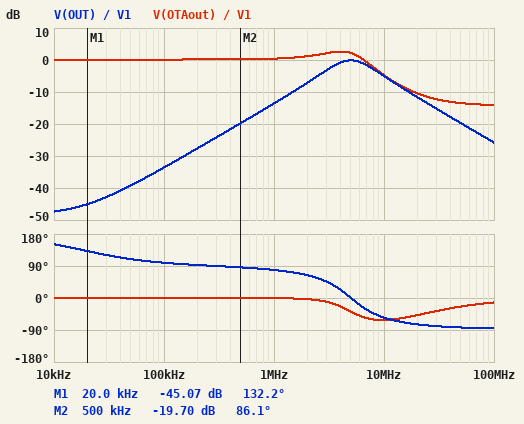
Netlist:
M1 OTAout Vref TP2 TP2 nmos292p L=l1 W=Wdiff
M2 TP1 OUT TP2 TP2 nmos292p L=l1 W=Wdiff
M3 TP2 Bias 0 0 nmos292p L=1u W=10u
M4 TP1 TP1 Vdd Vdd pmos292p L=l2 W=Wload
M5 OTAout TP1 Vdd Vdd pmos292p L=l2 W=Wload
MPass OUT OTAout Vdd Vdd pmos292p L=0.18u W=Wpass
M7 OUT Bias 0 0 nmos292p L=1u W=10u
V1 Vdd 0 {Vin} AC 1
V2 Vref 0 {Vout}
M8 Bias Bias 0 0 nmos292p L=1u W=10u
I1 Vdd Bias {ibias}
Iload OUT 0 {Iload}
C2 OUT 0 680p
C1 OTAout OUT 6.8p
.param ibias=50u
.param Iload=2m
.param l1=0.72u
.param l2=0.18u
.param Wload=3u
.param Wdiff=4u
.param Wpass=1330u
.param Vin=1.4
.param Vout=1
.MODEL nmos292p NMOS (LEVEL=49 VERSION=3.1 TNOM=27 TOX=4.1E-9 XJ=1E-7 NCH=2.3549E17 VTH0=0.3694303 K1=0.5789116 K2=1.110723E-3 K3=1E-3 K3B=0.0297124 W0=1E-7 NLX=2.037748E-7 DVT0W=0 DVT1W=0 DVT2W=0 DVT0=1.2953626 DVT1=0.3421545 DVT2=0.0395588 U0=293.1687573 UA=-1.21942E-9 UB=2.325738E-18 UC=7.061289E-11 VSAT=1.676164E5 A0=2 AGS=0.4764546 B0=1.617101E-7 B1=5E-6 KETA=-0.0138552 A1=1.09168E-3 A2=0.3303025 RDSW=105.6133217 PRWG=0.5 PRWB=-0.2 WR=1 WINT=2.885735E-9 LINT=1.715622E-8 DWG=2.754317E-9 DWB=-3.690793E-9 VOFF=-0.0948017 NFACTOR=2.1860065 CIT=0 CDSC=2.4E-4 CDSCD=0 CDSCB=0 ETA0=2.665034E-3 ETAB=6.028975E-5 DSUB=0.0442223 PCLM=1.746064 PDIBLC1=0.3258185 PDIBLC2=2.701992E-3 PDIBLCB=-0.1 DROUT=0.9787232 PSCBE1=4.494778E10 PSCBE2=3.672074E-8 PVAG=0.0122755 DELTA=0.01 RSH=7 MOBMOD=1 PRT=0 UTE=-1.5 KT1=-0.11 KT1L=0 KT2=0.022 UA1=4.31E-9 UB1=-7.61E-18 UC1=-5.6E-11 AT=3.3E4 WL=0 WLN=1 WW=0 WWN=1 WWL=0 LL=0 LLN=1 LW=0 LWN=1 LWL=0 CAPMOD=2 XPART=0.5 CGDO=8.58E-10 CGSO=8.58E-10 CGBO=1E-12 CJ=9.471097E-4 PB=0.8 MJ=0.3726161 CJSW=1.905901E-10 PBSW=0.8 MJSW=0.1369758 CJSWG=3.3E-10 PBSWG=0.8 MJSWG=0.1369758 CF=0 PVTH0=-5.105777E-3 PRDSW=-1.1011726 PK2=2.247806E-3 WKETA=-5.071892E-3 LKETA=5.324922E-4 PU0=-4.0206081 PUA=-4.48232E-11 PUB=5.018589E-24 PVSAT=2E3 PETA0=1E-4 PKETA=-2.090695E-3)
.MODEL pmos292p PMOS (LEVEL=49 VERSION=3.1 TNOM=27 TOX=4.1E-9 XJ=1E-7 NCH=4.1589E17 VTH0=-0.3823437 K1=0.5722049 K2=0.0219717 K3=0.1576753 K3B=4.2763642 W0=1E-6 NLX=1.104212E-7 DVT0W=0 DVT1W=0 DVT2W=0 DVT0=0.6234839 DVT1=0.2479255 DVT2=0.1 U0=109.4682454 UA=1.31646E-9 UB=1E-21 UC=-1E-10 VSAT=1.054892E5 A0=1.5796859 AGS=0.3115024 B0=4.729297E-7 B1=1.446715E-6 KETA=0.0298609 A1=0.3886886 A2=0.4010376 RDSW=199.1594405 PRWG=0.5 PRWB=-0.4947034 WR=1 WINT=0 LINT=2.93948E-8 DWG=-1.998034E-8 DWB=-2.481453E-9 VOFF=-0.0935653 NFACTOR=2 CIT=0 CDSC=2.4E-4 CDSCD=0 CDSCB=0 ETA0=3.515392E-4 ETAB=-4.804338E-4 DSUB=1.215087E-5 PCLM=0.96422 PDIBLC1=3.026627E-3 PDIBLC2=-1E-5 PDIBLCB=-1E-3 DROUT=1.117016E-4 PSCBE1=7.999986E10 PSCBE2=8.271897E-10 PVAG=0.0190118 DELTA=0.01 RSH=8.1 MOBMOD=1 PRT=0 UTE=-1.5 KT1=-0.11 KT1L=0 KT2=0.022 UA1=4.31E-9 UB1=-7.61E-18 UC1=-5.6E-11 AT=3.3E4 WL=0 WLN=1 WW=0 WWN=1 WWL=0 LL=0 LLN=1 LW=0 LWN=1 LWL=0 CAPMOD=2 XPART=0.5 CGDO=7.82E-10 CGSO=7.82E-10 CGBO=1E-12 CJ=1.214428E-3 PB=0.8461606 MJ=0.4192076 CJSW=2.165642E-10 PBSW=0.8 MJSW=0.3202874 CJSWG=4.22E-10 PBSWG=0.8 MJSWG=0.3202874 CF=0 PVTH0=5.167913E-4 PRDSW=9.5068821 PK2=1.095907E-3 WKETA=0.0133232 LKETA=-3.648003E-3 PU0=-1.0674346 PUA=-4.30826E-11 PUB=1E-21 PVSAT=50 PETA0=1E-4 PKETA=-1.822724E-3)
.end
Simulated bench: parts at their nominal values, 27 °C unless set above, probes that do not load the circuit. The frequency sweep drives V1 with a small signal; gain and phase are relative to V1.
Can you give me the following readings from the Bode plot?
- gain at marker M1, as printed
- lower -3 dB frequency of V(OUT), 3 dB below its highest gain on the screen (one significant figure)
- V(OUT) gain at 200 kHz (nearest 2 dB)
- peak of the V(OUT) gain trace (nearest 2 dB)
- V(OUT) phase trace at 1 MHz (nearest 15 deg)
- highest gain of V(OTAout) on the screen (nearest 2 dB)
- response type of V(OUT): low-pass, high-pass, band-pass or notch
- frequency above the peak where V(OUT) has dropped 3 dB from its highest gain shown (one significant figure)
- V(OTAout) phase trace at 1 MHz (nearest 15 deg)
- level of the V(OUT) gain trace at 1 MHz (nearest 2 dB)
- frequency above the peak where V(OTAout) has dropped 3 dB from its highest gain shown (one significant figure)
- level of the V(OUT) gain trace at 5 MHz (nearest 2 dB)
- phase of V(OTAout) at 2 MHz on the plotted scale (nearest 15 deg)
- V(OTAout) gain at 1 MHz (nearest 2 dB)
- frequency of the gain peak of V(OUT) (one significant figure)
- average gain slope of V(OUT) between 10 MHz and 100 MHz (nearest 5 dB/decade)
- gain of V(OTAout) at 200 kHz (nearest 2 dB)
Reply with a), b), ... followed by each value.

a) -45.07 dB
b) 3 MHz
c) -28 dB
d) 0 dB
e) 75 deg
f) 2 dB
g) band-pass
h) 8 MHz
i) 0 deg
j) -14 dB
k) 7 MHz
l) 0 dB
m) 0 deg
n) 0 dB
o) 5 MHz
p) -20 dB/decade
q) 0 dB
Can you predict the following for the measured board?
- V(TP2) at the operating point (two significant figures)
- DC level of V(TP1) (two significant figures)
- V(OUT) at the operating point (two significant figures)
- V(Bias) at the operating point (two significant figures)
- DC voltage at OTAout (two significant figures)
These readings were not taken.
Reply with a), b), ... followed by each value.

a) 380 mV
b) 750 mV
c) 1.0 V
d) 620 mV
e) 840 mV
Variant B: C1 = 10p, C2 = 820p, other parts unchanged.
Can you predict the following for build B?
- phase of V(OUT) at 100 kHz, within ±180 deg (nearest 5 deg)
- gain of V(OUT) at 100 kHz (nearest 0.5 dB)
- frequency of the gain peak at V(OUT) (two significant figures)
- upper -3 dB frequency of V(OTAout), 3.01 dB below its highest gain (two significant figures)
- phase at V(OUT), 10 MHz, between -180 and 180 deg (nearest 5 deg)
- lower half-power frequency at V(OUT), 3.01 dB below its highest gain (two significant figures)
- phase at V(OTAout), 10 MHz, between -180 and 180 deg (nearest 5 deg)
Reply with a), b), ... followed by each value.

a) 95 deg
b) -30.5 dB
c) 3.9 MHz
d) 5.6 MHz
e) -60 deg
f) 2.3 MHz
g) -65 deg
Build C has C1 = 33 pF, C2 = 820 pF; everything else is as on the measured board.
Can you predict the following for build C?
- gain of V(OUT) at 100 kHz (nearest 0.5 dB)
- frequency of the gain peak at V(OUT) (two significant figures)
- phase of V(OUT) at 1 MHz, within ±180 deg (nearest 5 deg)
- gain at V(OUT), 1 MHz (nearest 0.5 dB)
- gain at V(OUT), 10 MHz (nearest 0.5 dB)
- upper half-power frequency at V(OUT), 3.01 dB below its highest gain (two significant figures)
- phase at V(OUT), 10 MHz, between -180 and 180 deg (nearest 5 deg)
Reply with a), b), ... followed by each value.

a) -21.0 dB
b) 2.4 MHz
c) 45 deg
d) -2.5 dB
e) -6.5 dB
f) 5.9 MHz
g) -60 deg
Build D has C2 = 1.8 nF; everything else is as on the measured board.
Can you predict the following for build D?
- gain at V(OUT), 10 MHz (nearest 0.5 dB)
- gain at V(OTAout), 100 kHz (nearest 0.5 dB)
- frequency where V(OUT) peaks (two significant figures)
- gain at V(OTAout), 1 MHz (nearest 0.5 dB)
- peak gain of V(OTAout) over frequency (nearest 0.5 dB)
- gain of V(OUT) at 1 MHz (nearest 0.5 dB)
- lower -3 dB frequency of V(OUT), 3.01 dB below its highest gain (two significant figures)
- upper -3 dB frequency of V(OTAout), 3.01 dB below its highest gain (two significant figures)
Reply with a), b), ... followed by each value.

a) -13.5 dB
b) 0 dB
c) 3.1 MHz
d) 1.0 dB
e) 4.5 dB
f) -13.0 dB
g) 2.2 MHz
h) 3.7 MHz
